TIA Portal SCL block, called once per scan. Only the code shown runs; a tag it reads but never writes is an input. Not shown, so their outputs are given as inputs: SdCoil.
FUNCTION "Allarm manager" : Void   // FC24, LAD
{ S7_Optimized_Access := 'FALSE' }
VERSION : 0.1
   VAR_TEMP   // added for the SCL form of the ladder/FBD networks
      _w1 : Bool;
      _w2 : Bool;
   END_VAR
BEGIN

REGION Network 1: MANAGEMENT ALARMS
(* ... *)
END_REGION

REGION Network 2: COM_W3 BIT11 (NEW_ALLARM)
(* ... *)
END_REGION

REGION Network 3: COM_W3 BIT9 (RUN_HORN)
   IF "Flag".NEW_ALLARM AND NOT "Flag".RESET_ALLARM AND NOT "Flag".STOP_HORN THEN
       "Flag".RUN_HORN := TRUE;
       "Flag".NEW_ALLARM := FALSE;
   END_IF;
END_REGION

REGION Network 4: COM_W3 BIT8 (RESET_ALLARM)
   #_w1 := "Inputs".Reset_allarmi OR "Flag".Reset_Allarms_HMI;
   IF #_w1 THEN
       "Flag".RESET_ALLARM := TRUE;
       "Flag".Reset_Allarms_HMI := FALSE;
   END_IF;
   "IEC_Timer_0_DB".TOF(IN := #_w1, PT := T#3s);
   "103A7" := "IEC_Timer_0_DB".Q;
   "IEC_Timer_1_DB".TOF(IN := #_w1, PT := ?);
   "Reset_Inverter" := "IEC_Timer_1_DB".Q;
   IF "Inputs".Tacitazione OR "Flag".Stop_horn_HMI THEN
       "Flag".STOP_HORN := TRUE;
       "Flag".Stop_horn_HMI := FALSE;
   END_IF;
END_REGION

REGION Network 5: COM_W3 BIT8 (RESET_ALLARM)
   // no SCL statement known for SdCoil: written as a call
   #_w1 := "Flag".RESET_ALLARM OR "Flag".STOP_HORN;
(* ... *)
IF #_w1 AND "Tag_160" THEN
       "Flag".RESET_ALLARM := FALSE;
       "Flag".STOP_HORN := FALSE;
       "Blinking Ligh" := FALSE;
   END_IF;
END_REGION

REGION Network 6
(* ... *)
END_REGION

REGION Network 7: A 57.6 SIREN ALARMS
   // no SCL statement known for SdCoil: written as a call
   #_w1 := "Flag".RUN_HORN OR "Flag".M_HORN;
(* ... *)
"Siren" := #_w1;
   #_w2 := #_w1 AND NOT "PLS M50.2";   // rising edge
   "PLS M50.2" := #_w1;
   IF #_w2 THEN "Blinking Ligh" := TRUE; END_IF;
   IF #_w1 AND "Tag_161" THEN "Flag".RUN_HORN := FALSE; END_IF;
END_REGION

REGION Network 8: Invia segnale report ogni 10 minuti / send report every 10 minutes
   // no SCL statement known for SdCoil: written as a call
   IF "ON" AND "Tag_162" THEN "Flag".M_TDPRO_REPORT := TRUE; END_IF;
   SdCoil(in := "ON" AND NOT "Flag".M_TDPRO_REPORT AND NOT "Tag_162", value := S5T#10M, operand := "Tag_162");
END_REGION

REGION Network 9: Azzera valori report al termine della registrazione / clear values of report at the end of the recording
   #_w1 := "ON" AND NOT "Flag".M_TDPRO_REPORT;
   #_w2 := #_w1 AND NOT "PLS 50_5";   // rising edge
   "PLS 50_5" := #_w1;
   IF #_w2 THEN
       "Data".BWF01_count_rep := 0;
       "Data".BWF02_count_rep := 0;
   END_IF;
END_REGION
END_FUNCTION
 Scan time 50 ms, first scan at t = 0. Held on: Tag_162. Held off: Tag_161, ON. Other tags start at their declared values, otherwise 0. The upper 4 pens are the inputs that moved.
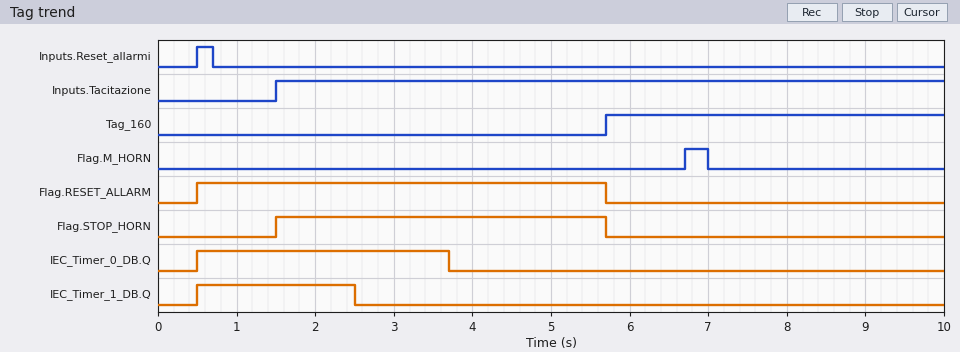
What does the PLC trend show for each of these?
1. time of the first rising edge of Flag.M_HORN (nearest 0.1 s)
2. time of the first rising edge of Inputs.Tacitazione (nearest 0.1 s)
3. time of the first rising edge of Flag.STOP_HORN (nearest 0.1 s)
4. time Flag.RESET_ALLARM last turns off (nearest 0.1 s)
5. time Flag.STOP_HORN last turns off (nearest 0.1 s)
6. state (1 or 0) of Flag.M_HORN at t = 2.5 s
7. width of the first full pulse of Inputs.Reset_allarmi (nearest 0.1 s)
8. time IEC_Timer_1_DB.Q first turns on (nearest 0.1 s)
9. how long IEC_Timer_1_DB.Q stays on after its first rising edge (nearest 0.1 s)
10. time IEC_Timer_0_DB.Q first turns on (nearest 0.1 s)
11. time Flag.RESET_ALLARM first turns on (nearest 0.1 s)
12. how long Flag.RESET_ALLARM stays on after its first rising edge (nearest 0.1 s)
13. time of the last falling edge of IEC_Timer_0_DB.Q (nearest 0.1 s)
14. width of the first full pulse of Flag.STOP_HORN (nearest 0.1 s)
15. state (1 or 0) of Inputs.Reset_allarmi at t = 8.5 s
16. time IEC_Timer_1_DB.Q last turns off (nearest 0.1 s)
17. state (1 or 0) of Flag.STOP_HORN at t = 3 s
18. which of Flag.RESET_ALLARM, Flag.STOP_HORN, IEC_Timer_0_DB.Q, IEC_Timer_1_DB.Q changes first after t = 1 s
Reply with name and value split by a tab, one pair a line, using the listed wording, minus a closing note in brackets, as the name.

time of the first rising edge of Flag.M_HORN	6.7 s
time of the first rising edge of Inputs.Tacitazione	1.5 s
time of the first rising edge of Flag.STOP_HORN	1.5 s
time Flag.RESET_ALLARM last turns off	5.7 s
time Flag.STOP_HORN last turns off	5.7 s
state (1 or 0) of Flag.M_HORN at t = 2.5 s	0
width of the first full pulse of Inputs.Reset_allarmi	0.2 s
time IEC_Timer_1_DB.Q first turns on	0.5 s
how long IEC_Timer_1_DB.Q stays on after its first rising edge	2.0 s
time IEC_Timer_0_DB.Q first turns on	0.5 s
time Flag.RESET_ALLARM first turns on	0.5 s
how long Flag.RESET_ALLARM stays on after its first rising edge	5.2 s
time of the last falling edge of IEC_Timer_0_DB.Q	3.7 s
width of the first full pulse of Flag.STOP_HORN	4.2 s
state (1 or 0) of Inputs.Reset_allarmi at t = 8.5 s	0
time IEC_Timer_1_DB.Q last turns off	2.5 s
state (1 or 0) of Flag.STOP_HORN at t = 3 s	1
which of Flag.RESET_ALLARM, Flag.STOP_HORN, IEC_Timer_0_DB.Q, IEC_Timer_1_DB.Q changes first after t = 1 s	Flag.STOP_HORN
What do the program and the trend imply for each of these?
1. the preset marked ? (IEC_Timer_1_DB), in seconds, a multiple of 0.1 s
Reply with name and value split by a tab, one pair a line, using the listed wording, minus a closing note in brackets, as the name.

the preset marked ? (IEC_Timer_1_DB), in seconds, a multiple of 0.1 s	1.8 s
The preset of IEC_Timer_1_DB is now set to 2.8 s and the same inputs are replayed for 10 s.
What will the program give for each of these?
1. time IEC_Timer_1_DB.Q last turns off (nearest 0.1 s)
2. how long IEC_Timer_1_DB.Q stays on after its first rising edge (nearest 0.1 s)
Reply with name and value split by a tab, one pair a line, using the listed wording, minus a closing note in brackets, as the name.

time IEC_Timer_1_DB.Q last turns off	3.5 s
how long IEC_Timer_1_DB.Q stays on after its first rising edge	3.0 s
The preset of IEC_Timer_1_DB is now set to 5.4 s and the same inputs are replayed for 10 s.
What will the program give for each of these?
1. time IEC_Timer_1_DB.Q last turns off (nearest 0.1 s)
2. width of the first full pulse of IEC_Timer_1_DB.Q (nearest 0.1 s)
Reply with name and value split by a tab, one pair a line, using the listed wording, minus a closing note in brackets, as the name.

time IEC_Timer_1_DB.Q last turns off	6.1 s
width of the first full pulse of IEC_Timer_1_DB.Q	5.6 s
